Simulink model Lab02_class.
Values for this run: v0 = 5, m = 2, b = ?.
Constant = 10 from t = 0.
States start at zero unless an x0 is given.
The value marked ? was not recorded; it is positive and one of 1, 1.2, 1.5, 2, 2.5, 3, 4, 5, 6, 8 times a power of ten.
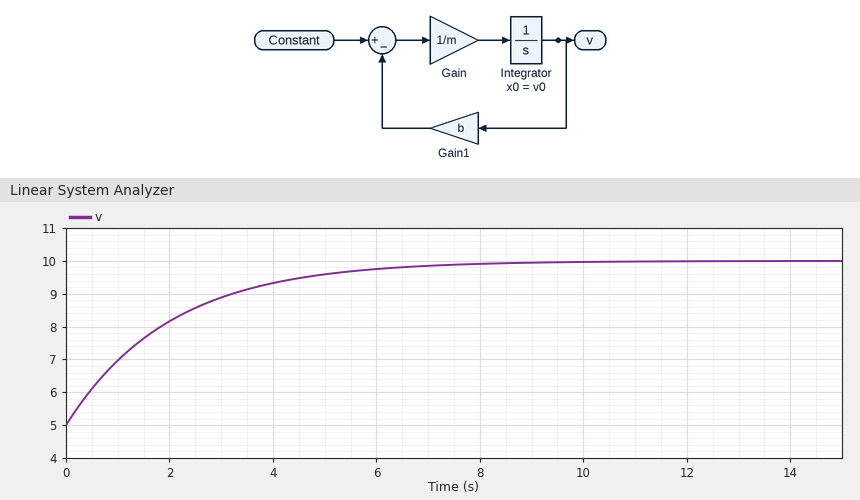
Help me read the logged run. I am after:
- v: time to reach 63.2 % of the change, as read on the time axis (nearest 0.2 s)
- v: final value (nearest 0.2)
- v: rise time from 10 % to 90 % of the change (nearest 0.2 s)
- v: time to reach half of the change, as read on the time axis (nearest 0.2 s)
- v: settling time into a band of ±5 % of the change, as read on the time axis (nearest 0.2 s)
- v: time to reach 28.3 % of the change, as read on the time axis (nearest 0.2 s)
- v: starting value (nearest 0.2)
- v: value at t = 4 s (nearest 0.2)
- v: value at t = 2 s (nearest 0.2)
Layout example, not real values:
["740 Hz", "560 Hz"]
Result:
["2.0 s", "10.0", "4.4 s", "1.4 s", "6.0 s", "0.6 s", "5.0", "9.4", "8.2"]
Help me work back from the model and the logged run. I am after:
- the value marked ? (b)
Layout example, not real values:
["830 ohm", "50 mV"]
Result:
["1"]
